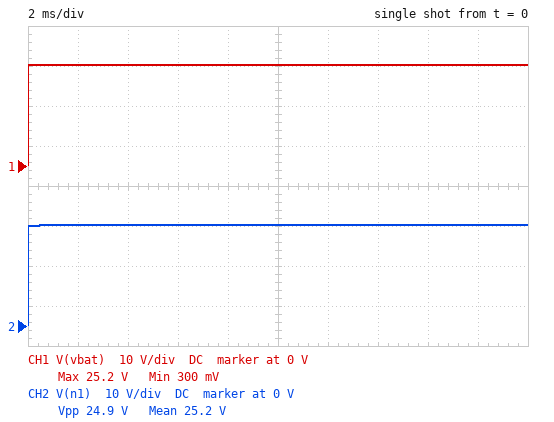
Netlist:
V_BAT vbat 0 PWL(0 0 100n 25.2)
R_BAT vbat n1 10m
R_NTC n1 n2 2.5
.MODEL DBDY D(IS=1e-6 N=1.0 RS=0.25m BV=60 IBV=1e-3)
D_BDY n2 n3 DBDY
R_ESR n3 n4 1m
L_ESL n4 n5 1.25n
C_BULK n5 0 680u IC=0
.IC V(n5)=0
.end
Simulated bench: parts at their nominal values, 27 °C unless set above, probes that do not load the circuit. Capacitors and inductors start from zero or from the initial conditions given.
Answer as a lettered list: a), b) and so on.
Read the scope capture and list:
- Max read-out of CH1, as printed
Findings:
a) 25.2 V
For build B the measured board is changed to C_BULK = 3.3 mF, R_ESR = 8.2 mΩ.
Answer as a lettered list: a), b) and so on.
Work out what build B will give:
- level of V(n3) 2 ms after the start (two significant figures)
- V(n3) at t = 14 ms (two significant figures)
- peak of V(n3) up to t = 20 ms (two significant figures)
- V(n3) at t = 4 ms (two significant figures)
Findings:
a) 5.4 V
b) 20 V
c) 23 V
d) 9.5 V
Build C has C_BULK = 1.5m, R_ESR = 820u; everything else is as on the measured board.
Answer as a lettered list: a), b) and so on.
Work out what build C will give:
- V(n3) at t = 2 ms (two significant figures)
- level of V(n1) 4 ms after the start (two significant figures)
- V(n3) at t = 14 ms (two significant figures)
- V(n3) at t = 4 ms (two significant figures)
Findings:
a) 10 V
b) 25 V
c) 24 V
d) 16 V
